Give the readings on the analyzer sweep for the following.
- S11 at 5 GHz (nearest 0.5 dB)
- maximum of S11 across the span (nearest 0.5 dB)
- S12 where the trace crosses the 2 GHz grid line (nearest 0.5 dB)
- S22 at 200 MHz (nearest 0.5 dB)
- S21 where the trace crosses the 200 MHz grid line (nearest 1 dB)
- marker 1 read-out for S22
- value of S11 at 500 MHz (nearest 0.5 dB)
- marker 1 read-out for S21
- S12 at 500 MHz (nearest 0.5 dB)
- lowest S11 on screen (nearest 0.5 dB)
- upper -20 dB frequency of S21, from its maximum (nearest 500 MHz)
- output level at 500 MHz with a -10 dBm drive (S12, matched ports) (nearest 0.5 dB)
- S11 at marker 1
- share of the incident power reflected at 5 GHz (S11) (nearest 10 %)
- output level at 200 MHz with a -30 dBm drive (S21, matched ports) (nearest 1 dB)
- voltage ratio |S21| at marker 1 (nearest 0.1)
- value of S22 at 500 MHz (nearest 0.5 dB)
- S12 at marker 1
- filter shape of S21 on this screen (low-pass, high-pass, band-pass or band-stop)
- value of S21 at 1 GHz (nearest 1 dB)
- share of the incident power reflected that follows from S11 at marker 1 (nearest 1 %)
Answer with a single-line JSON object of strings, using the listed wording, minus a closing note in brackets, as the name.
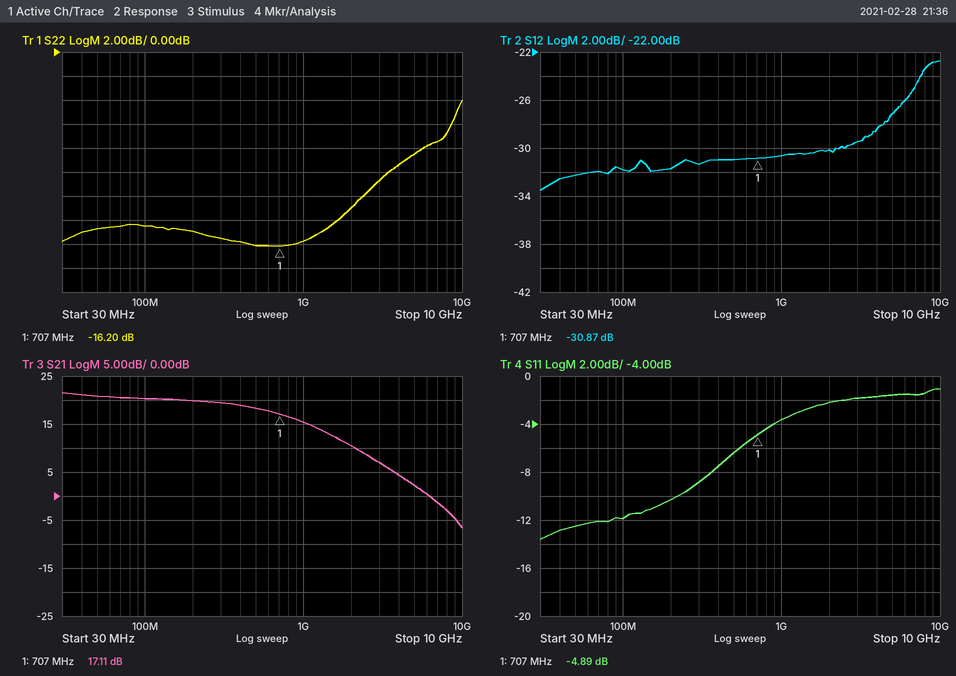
{"S11 at 5 GHz": "-1.5 dB", "maximum of S11 across the span": "-1.0 dB", "S12 where the trace crosses the 2 GHz grid line": "-30.0 dB", "S22 at 200 MHz": "-15.0 dB", "S21 where the trace crosses the 200 MHz grid line": "20 dB", "marker 1 read-out for S22": "-16.20 dB", "value of S11 at 500 MHz": "-6.5 dB", "marker 1 read-out for S21": "17.11 dB", "S12 at 500 MHz": "-31.0 dB", "lowest S11 on screen": "-13.5 dB", "upper -20 dB frequency of S21, from its maximum": "5.5 GHz", "output level at 500 MHz with a -10 dBm drive (S12, matched ports)": "-41.0 dBm", "S11 at marker 1": "-4.89 dB", "share of the incident power reflected at 5 GHz (S11)": "70 %", "output level at 200 MHz with a -30 dBm drive (S21, matched ports)": "-10 dBm", "voltage ratio |S21| at marker 1": "7.2", "value of S22 at 500 MHz": "-16.0 dB", "S12 at marker 1": "-30.87 dB", "filter shape of S21 on this screen": "low-pass", "value of S21 at 1 GHz": "15 dB", "share of the incident power reflected that follows from S11 at marker 1": "32 %"}
